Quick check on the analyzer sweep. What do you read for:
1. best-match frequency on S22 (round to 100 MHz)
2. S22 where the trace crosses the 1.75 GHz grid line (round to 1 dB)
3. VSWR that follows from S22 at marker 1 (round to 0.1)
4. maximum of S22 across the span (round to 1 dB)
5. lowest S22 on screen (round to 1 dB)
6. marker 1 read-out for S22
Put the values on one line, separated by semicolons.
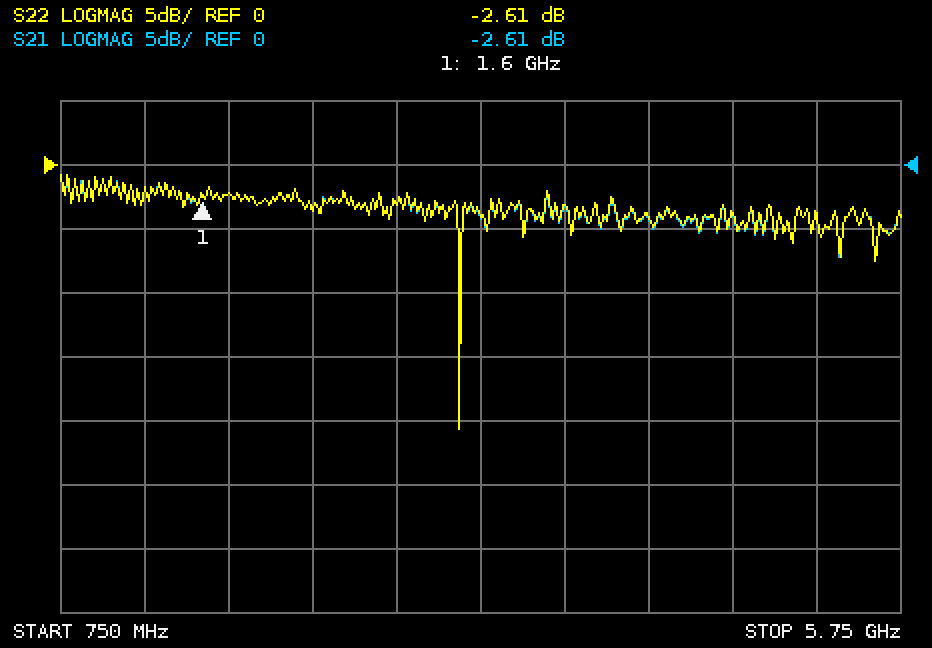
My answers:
3.1 GHz; -2 dB; 6.7; -1 dB; -21 dB; -2.61 dB
